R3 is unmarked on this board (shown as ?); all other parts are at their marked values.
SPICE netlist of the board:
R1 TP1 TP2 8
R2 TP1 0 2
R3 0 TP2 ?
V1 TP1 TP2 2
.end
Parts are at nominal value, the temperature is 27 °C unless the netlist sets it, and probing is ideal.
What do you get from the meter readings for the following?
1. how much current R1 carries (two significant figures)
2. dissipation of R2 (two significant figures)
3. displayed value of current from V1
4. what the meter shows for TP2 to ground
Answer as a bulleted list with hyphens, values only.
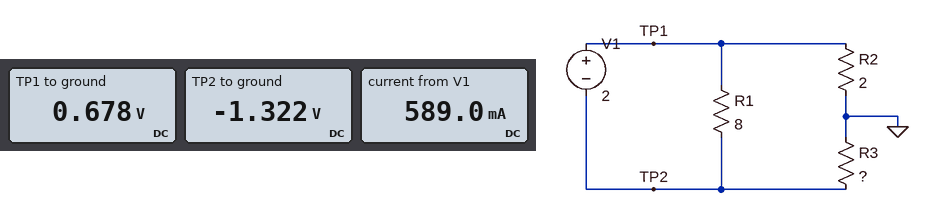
- 250 mA
- 230 mW
- 589.0 mA
- -1.322 V
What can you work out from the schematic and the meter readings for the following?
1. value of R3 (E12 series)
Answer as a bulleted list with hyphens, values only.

- 3.9 Ω
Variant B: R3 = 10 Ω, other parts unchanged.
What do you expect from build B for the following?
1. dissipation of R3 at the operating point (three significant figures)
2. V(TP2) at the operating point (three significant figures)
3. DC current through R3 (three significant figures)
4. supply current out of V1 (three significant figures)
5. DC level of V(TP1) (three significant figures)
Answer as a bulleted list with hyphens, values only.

- 278 mW
- -1.67 V
- 167 mA
- 417 mA
- 333 mV
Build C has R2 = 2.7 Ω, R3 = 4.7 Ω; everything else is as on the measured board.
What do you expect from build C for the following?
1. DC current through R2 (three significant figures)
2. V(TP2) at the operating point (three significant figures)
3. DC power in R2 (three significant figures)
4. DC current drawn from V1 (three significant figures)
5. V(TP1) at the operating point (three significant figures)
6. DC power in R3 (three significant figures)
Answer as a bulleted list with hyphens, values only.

- 270 mA
- -1.27 V
- 197 mW
- 520 mA
- 730 mV
- 343 mW
